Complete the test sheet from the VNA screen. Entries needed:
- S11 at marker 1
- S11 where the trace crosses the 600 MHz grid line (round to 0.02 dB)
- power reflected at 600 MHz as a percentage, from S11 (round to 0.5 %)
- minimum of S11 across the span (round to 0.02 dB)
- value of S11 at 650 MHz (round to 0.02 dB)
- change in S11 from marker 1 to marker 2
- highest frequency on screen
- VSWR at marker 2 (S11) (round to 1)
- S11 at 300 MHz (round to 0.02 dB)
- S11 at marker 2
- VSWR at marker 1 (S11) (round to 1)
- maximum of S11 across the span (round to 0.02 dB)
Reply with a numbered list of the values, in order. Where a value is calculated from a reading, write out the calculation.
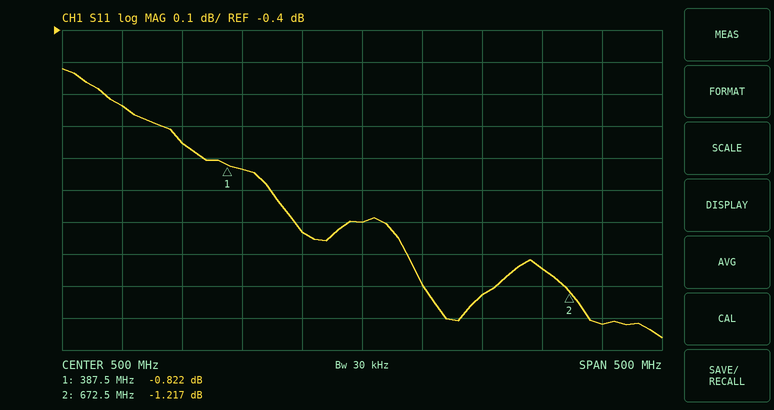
1. -0.822 dB
2. -1.22 dB
3. 10^(-1.22/10) ≈ 75.5 %
4. -1.36 dB
5. -1.14 dB
6. -1.217 − (-0.822) = -0.395 dB
7. 750 MHz
8. (1 + 0.8693)/(1 − 0.8693) ≈ 14
9. -0.64 dB
10. -1.217 dB
11. (1 + 0.9097)/(1 − 0.9097) ≈ 21
12. -0.52 dB
